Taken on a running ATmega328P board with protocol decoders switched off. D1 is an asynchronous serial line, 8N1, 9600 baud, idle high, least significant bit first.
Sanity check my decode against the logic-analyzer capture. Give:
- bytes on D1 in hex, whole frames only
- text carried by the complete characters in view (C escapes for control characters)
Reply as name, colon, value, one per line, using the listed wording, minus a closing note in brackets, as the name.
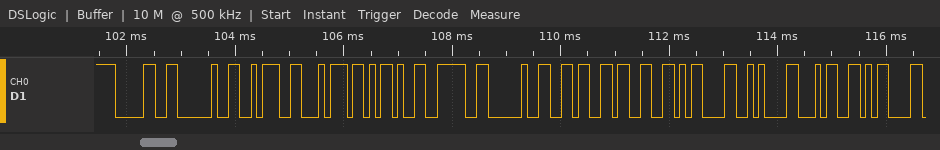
bytes on D1 in hex, whole frames only: 0x30 0x20 0x3A 0x74 0x2D 0x3E 0x20 0x36 0x33 0x0D 0x0A 0x34 0x0D
text carried by the complete characters in view: "0 :t-> 63\r\n4\r"
